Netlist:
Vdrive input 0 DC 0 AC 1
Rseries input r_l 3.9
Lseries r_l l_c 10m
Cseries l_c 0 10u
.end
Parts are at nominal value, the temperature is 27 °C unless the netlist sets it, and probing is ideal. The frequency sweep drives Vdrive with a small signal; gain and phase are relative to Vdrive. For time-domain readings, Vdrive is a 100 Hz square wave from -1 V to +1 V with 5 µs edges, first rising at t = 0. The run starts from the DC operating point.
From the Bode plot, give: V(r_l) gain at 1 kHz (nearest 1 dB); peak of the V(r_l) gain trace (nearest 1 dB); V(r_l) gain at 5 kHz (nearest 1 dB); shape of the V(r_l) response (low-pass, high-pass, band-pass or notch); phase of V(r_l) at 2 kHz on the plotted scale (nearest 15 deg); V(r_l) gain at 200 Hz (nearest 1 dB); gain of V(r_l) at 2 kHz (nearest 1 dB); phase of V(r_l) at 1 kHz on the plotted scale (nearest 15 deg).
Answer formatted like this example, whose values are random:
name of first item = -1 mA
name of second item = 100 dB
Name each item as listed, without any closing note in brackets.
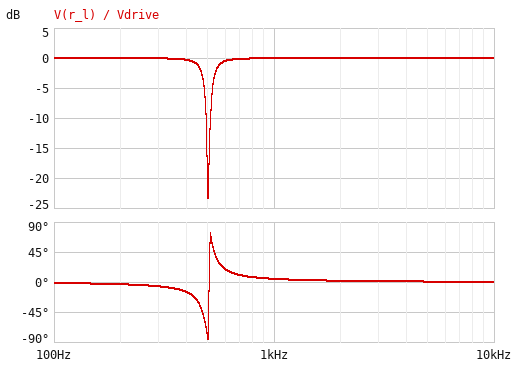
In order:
V(r_l) gain at 1 kHz = 0 dB
peak of the V(r_l) gain trace = 0 dB
V(r_l) gain at 5 kHz = 0 dB
shape of the V(r_l) response = notch
phase of V(r_l) at 2 kHz on the plotted scale = 0 deg
V(r_l) gain at 200 Hz = 0 dB
gain of V(r_l) at 2 kHz = 0 dB
phase of V(r_l) at 1 kHz on the plotted scale = 0 deg
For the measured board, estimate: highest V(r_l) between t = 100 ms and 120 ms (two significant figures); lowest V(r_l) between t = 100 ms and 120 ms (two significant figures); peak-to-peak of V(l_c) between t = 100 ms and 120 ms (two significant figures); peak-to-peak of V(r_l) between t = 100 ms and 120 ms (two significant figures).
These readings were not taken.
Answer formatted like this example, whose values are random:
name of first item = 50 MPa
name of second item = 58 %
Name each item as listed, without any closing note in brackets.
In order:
highest V(r_l) between t = 100 ms and 120 ms = 1.3 V
lowest V(r_l) between t = 100 ms and 120 ms = -1.3 V
peak-to-peak of V(l_c) between t = 100 ms and 120 ms = 7.3 V
peak-to-peak of V(r_l) between t = 100 ms and 120 ms = 2.6 V
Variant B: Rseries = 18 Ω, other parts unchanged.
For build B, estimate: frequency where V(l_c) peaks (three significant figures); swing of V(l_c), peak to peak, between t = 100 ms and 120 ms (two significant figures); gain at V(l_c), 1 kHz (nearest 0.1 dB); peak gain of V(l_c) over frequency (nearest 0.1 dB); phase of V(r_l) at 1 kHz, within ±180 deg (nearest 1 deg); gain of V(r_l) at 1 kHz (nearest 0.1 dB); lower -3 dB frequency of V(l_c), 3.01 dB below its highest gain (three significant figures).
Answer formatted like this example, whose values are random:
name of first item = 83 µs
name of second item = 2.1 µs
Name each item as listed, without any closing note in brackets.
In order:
frequency where V(l_c) peaks = 461 Hz
swing of V(l_c), peak to peak, between t = 100 ms and 120 ms = 3.6 V
gain at V(l_c), 1 kHz = -10.0 dB
peak gain of V(l_c) over frequency = 5.3 dB
phase of V(r_l) at 1 kHz, within ±180 deg = 21 deg
gain of V(r_l) at 1 kHz = -0.6 dB
lower -3 dB frequency of V(l_c), 3.01 dB below its highest gain = 272 Hz
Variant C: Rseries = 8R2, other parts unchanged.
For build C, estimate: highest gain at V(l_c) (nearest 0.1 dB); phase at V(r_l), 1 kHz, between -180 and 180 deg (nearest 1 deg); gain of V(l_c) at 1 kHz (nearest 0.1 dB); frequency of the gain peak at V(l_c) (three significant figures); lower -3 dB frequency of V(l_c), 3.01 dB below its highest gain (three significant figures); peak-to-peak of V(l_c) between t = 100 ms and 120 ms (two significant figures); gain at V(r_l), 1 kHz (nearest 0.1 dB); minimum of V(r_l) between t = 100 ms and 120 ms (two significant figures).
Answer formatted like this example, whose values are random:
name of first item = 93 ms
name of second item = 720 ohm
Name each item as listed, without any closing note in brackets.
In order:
highest gain at V(l_c) = 11.8 dB
phase at V(r_l), 1 kHz, between -180 and 180 deg = 10 deg
gain of V(l_c) at 1 kHz = -9.5 dB
frequency of the gain peak at V(l_c) = 495 Hz
lower -3 dB frequency of V(l_c), 3.01 dB below its highest gain = 424 Hz
peak-to-peak of V(l_c) between t = 100 ms and 120 ms = 5.0 V
gain at V(r_l), 1 kHz = -0.1 dB
minimum of V(r_l) between t = 100 ms and 120 ms = -1.3 V
